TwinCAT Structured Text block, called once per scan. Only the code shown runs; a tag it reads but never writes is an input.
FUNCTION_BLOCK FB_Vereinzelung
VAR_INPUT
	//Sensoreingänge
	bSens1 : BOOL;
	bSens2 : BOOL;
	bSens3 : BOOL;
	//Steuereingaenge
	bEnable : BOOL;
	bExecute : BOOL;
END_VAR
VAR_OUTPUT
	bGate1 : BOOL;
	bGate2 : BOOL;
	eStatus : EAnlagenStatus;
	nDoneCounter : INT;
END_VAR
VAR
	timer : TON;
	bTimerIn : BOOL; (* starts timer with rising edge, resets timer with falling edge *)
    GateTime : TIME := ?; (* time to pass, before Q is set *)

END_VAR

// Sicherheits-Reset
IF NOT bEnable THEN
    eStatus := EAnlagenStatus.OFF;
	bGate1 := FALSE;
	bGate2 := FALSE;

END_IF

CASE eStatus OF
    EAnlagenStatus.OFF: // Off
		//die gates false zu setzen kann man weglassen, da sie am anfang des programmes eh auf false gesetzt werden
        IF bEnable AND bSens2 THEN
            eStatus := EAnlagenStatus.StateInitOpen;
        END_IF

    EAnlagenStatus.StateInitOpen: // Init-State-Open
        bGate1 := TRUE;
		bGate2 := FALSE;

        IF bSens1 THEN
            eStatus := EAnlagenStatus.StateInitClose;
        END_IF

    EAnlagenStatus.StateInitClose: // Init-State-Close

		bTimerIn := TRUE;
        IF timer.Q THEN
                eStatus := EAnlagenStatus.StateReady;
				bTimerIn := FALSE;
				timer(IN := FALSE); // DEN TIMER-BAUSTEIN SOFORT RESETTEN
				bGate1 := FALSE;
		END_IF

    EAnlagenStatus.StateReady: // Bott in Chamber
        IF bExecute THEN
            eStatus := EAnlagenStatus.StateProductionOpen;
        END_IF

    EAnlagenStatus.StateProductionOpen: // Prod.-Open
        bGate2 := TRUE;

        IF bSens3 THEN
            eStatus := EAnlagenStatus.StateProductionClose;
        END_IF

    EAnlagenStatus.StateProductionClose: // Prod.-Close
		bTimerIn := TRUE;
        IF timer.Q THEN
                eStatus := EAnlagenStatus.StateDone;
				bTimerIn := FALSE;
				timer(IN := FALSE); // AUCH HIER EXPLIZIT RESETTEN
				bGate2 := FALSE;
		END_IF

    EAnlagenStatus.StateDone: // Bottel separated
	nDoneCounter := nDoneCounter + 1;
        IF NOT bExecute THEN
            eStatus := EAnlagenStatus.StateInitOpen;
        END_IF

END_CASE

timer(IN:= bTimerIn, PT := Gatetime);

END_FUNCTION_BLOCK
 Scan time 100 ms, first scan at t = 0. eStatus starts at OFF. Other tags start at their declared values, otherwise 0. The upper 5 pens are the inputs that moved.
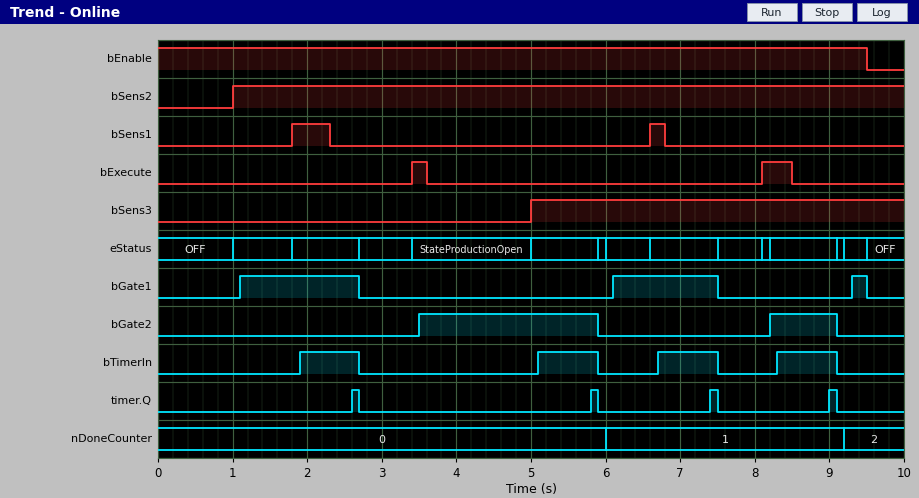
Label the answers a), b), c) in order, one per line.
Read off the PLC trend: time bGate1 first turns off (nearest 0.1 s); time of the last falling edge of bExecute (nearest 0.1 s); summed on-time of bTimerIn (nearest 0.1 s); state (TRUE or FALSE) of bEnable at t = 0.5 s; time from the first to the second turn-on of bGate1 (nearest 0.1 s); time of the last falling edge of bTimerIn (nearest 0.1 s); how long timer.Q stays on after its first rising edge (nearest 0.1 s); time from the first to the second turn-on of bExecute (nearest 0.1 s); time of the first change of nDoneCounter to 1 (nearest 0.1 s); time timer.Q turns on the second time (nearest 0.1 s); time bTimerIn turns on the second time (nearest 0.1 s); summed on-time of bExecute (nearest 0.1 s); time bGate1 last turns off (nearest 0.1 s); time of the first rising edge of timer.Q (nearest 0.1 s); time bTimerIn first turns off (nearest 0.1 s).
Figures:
a) 2.7 s
b) 8.5 s
c) 3.2 s
d) TRUE
e) 5.0 s
f) 9.1 s
g) 0.1 s
h) 4.7 s
i) 6.0 s
j) 5.8 s
k) 5.1 s
l) 0.6 s
m) 9.5 s
n) 2.6 s
o) 2.7 s
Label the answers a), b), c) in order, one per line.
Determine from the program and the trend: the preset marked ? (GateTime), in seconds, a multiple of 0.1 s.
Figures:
a) 0.7 s
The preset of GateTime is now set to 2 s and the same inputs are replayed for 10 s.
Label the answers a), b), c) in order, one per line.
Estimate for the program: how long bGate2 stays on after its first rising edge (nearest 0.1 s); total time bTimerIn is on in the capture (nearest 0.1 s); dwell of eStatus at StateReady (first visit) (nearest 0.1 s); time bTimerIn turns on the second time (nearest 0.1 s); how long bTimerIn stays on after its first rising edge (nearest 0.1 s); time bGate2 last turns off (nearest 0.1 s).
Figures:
a) 1.3 s
b) 3.8 s
c) 4.1 s
d) 8.3 s
e) 2.1 s
f) 9.5 s
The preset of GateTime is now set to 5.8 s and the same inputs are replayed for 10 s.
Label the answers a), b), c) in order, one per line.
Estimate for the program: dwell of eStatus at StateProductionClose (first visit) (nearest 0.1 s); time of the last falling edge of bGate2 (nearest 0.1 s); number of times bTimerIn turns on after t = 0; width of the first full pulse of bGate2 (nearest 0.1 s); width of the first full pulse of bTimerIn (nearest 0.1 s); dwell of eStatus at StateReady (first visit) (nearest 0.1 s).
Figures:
a) 1.3 s
b) 9.5 s
c) 2
d) 1.3 s
e) 5.9 s
f) 0.3 s
